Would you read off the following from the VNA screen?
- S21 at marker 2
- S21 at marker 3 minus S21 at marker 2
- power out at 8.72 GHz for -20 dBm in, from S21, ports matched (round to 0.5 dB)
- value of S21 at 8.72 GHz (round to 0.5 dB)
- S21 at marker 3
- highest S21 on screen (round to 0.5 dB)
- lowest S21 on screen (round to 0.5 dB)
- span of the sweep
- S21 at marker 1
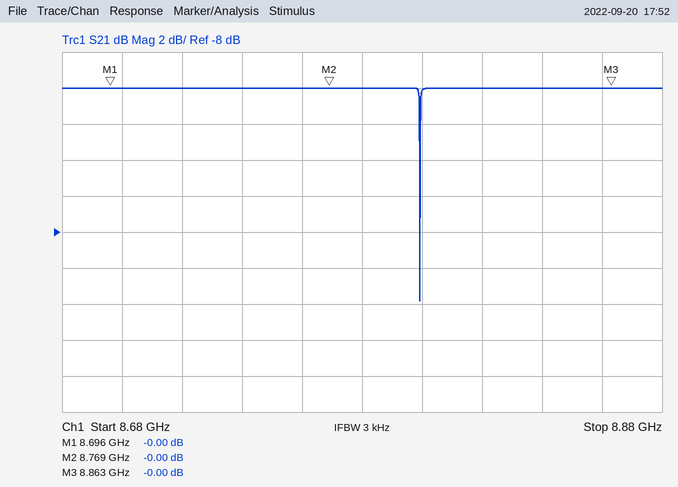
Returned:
-0.00 dB
0.00 dB
-20.0 dBm
0.0 dB
-0.00 dB
0.0 dB
-12.0 dB
200 MHz
-0.00 dB
